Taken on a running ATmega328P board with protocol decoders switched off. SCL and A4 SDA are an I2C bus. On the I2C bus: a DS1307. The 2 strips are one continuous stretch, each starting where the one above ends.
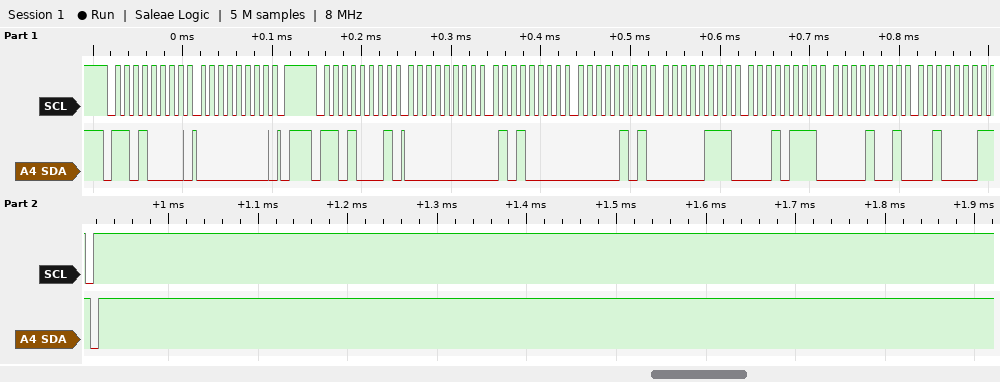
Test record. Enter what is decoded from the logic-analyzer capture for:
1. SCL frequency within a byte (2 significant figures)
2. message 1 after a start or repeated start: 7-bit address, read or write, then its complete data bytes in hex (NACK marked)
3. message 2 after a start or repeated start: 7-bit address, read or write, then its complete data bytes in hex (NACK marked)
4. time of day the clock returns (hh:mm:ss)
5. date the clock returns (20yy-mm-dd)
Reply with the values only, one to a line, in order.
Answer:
100 kHz
0x68 write: 00
0x68 read: 00 50 05 07 17 09 21 NACK
05:50:00
2021-09-17
